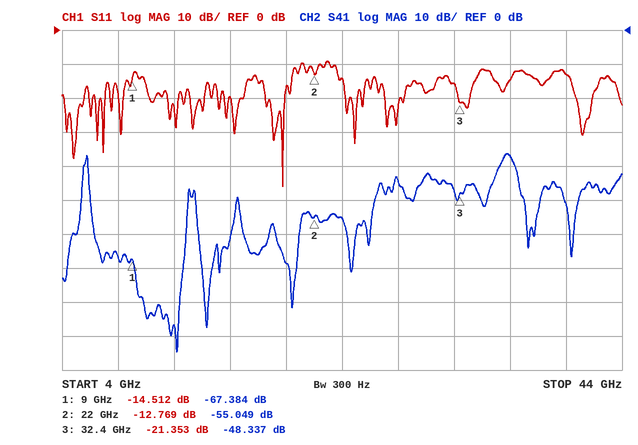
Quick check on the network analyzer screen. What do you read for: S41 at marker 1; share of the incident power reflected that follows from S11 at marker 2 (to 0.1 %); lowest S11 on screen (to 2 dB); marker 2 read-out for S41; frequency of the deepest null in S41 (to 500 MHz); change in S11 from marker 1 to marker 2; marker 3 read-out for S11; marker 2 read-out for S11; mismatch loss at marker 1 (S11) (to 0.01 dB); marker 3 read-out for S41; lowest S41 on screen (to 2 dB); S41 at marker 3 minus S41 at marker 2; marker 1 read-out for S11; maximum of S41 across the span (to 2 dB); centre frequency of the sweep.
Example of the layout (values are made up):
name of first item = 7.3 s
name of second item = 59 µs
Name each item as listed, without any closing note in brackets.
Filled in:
S41 at marker 1 = -67.384 dB
share of the incident power reflected that follows from S11 at marker 2 = 5.3 %
lowest S11 on screen = -46 dB
marker 2 read-out for S41 = -55.049 dB
frequency of the deepest null in S41 = 12.0 GHz
change in S11 from marker 1 to marker 2 = 1.743 dB
marker 3 read-out for S11 = -21.353 dB
marker 2 read-out for S11 = -12.769 dB
mismatch loss at marker 1 (S11) = 0.16 dB
marker 3 read-out for S41 = -48.337 dB
lowest S41 on screen = -94 dB
S41 at marker 3 minus S41 at marker 2 = 6.712 dB
marker 1 read-out for S11 = -14.512 dB
maximum of S41 across the span = -36 dB
centre frequency of the sweep = 24 GHz
